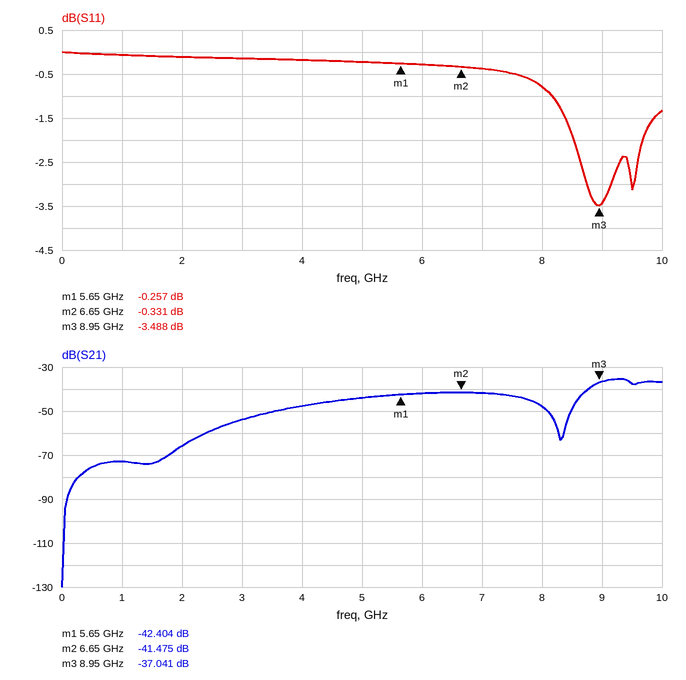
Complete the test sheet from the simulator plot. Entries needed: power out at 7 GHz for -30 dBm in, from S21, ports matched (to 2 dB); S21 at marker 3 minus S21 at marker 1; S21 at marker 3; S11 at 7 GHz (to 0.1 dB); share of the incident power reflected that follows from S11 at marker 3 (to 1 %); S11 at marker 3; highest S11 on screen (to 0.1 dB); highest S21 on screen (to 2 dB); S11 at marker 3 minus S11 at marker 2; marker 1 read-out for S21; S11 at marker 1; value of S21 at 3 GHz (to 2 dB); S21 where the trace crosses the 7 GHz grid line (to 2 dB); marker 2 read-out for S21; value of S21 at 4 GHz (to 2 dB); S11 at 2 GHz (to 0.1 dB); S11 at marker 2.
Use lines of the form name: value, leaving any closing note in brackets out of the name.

power out at 7 GHz for -30 dBm in, from S21, ports matched: -72 dBm
S21 at marker 3 minus S21 at marker 1: 5.363 dB
S21 at marker 3: -37.041 dB
S11 at 7 GHz: -0.4 dB
share of the incident power reflected that follows from S11 at marker 3: 45 %
S11 at marker 3: -3.488 dB
highest S11 on screen: 0.0 dB
highest S21 on screen: -36 dB
S11 at marker 3 minus S11 at marker 2: -3.157 dB
marker 1 read-out for S21: -42.404 dB
S11 at marker 1: -0.257 dB
value of S21 at 3 GHz: -54 dB
S21 where the trace crosses the 7 GHz grid line: -42 dB
marker 2 read-out for S21: -41.475 dB
value of S21 at 4 GHz: -48 dB
S11 at 2 GHz: -0.1 dB
S11 at marker 2: -0.331 dB
